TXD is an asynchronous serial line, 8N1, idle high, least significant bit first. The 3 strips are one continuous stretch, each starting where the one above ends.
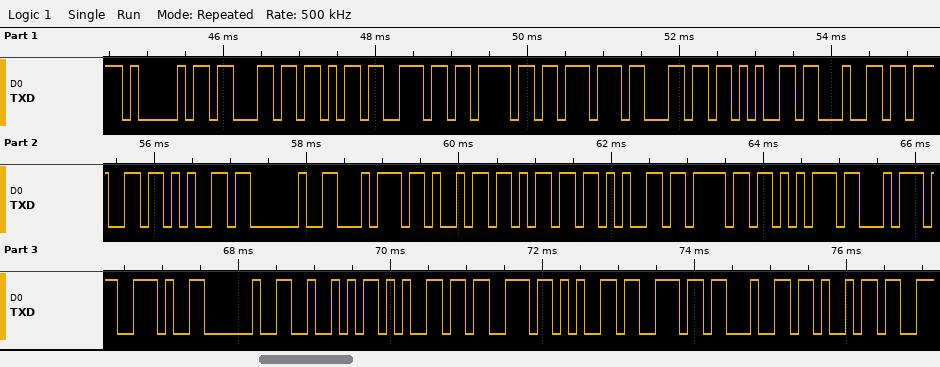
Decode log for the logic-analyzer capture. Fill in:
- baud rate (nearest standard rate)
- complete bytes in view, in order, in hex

9600 baud
41 63 6B 6E 6F 77 6C 65 64 67 65 20 74 69 6D 65 6F 75 74 2E 20 52 65 73 65 6E 64 69
